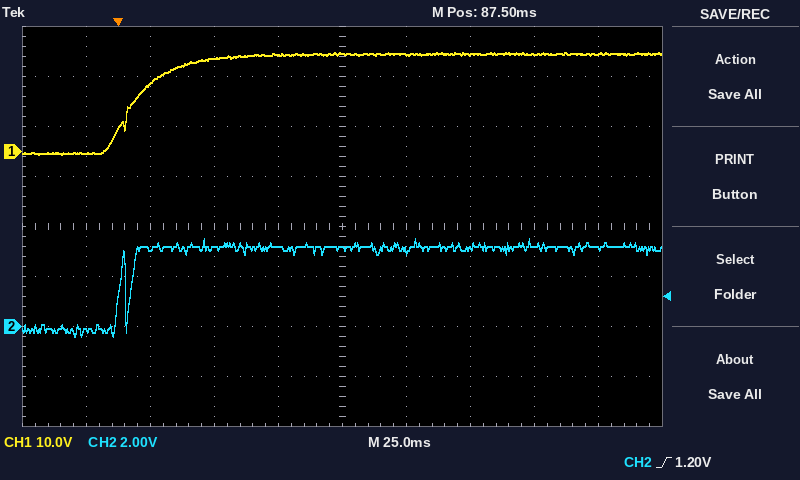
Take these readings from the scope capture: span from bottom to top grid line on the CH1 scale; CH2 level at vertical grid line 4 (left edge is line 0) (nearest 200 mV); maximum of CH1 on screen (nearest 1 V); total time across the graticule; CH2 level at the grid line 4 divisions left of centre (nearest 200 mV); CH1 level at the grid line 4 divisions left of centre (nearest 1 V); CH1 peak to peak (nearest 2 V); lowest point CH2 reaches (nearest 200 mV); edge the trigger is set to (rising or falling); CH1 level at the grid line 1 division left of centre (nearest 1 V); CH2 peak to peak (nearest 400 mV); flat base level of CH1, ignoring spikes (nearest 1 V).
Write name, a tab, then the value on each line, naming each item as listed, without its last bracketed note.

span from bottom to top grid line on the CH1 scale	80 V
CH2 level at vertical grid line 4 (left edge is line 0)	3.2 V
maximum of CH1 on screen	20 V
total time across the graticule	250 ms
CH2 level at the grid line 4 divisions left of centre	-200 mV
CH1 level at the grid line 4 divisions left of centre	0 V
CH1 peak to peak	20 V
lowest point CH2 reaches	-400 mV
edge the trigger is set to	rising
CH1 level at the grid line 1 division left of centre	19 V
CH2 peak to peak	4.0 V
flat base level of CH1, ignoring spikes	0 V
